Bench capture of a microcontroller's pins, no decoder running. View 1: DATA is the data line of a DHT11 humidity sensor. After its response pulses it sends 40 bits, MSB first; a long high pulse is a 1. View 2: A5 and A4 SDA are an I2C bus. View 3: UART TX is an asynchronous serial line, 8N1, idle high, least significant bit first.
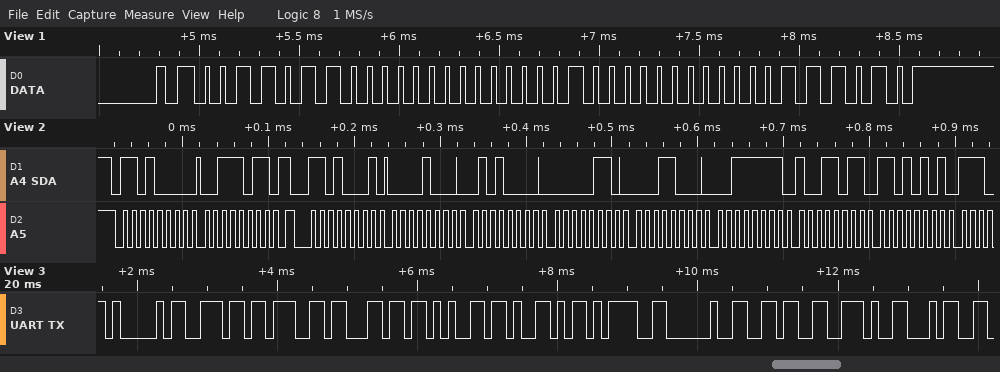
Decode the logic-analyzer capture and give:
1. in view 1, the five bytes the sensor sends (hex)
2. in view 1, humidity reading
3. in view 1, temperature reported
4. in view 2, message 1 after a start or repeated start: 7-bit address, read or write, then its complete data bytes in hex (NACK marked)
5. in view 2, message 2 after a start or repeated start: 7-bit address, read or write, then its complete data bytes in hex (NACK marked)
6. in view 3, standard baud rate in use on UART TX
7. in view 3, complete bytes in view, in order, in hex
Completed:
36 00 04 00 3A
54 %
4.0 °C
0x68 write: 3B
0x68 read: 08 50 06 18 3F 9B D5
9600 baud
41 6E 67 6C 65 59 3D 20 36 2E 34
